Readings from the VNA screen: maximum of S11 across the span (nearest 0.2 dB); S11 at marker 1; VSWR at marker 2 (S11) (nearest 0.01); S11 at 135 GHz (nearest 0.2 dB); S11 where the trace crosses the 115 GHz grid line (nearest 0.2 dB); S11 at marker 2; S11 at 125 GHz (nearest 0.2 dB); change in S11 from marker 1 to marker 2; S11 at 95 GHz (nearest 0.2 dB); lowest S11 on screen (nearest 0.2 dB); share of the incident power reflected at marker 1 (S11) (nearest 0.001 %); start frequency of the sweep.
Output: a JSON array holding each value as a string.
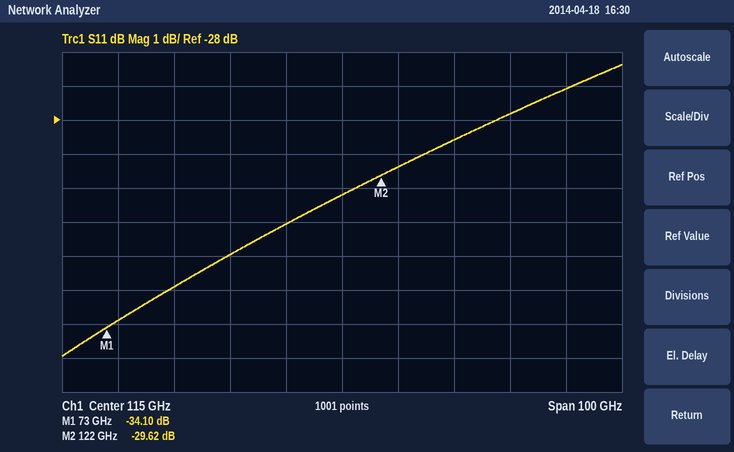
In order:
["-26.4 dB", "-34.10 dB", "1.07", "-28.6 dB", "-30.2 dB", "-29.62 dB", "-29.4 dB", "4.48 dB", "-32.0 dB", "-35.0 dB", "0.039 %", "65 GHz"]
